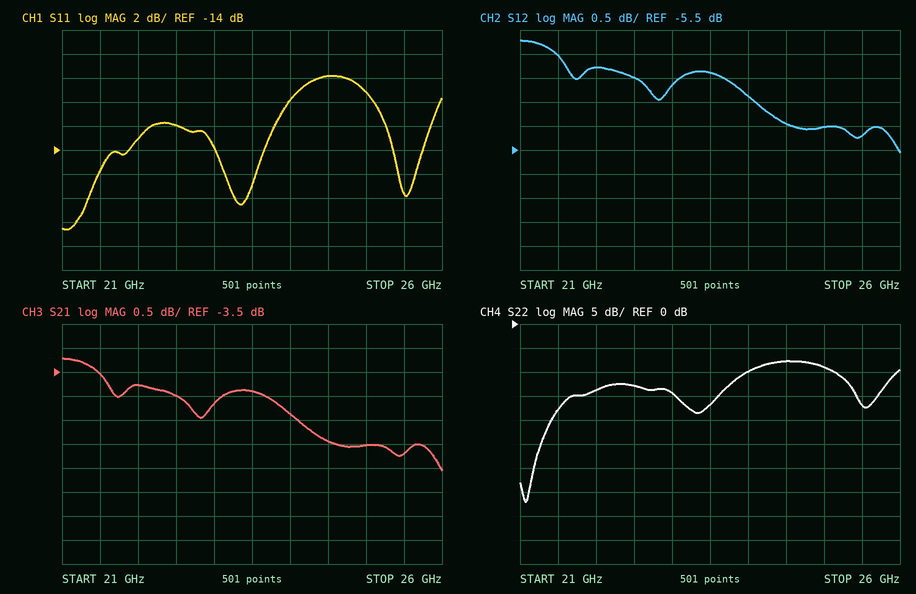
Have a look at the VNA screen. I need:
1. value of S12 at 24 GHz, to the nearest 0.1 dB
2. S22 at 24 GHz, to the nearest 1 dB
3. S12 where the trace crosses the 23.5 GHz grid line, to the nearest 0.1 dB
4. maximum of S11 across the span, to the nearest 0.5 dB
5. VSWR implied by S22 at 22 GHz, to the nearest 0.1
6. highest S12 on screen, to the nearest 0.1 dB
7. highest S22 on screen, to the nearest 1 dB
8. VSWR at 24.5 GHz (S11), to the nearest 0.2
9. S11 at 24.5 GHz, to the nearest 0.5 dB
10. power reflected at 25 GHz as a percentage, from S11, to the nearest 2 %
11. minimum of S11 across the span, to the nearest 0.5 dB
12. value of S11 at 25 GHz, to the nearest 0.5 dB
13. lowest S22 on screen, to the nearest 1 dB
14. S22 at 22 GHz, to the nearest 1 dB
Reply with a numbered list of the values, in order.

1. -4.4 dB
2. -10 dB
3. -3.9 dB
4. -8.0 dB
5. 1.5
6. -3.2 dB
7. -8 dB
8. 2.4
9. -8.0 dB
10. 12 %
11. -20.5 dB
12. -9.0 dB
13. -37 dB
14. -14 dB
